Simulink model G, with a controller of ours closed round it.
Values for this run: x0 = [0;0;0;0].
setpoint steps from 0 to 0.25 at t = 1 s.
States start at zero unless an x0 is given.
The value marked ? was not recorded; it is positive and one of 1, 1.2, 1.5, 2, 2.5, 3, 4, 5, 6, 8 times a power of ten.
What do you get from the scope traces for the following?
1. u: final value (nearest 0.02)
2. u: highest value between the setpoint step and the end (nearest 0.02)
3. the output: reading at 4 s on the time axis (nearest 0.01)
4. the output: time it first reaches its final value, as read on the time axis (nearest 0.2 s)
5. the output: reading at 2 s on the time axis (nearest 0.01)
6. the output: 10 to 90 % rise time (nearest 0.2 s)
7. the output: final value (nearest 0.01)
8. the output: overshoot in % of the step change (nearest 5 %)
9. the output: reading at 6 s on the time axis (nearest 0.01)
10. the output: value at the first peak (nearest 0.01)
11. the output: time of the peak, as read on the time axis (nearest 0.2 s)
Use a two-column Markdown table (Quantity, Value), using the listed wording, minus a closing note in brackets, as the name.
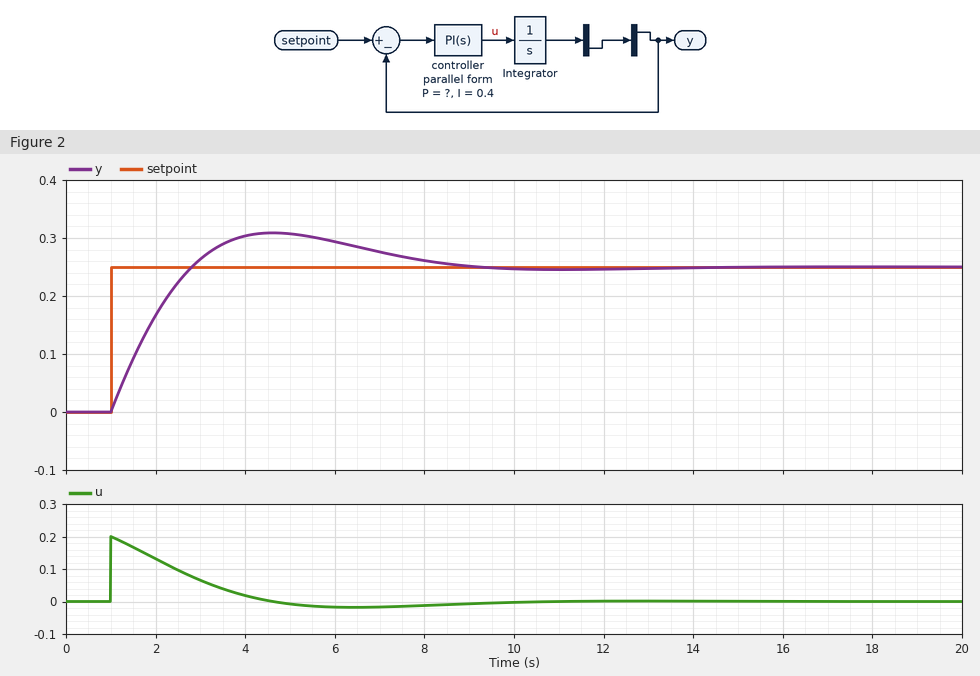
| Quantity | Value |
|---|---|
| u: final value | 0.00 |
| u: highest value between the setpoint step and the end | 0.20 |
| the output: reading at 4 s on the time axis | 0.30 |
| the output: time it first reaches its final value, as read on the time axis | 2.8 s |
| the output: reading at 2 s on the time axis | 0.17 |
| the output: 10 to 90 % rise time | 1.4 s |
| the output: final value | 0.25 |
| the output: overshoot in % of the step change | 25 % |
| the output: reading at 6 s on the time axis | 0.29 |
| the output: value at the first peak | 0.31 |
| the output: time of the peak, as read on the time axis | 4.6 s |
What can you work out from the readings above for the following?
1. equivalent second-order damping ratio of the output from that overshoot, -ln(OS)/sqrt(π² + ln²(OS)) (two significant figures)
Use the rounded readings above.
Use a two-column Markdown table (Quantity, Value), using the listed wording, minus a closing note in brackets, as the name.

| Quantity | Value |
|---|---|
| equivalent second-order damping ratio of the output from that overshoot, -ln(OS)/sqrt(π² + ln²(OS)) | 0.40 |
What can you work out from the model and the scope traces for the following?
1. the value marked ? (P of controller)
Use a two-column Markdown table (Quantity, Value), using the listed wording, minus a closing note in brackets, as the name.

| Quantity | Value |
|---|---|
| the value marked ? | 0.8 |
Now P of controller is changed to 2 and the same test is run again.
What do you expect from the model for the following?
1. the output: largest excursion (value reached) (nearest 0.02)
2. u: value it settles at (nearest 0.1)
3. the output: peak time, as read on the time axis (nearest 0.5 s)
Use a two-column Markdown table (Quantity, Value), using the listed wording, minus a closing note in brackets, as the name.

| Quantity | Value |
|---|---|
| the output: largest excursion (value reached) | 0.26 |
| u: value it settles at | 0.0 |
| the output: peak time, as read on the time axis | 3.5 s |
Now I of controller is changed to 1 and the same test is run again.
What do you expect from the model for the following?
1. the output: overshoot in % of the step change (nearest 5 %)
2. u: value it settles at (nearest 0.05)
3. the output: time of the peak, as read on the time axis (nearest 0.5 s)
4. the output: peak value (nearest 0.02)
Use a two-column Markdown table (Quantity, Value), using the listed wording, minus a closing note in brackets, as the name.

| Quantity | Value |
|---|---|
| the output: overshoot in % of the step change | 35 % |
| u: value it settles at | 0.00 |
| the output: time of the peak, as read on the time axis | 3.5 s |
| the output: peak value | 0.34 |
